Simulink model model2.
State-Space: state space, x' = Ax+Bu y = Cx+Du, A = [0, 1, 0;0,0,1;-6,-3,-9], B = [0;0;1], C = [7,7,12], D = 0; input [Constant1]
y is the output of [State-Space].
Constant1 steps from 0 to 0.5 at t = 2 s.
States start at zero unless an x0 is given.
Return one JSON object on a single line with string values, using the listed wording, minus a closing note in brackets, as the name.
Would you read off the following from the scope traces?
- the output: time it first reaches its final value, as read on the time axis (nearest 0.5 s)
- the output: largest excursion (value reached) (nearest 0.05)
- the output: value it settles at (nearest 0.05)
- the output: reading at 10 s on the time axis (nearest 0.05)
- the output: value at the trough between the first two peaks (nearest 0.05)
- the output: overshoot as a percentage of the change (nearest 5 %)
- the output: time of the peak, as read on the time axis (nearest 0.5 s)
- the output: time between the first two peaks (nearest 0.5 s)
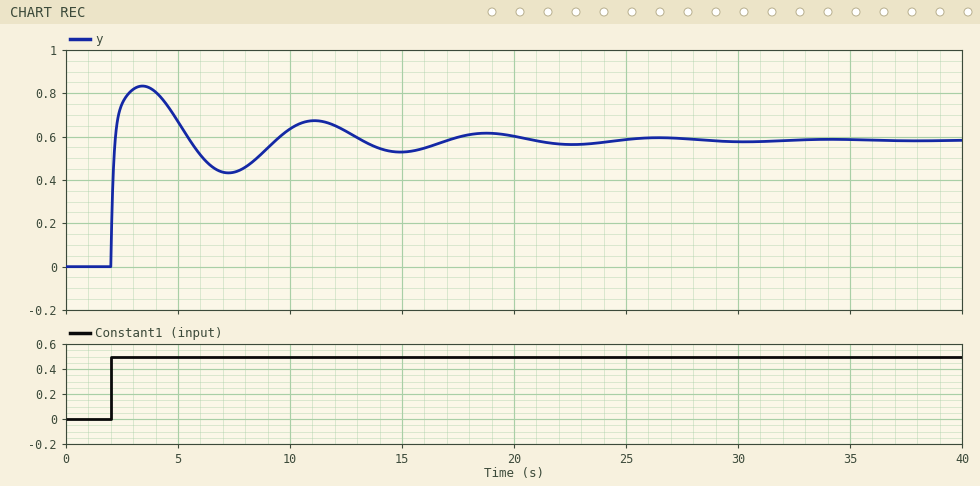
{"the output: time it first reaches its final value, as read on the time axis": "2.0 s", "the output: largest excursion (value reached)": "0.85", "the output: value it settles at": "0.60", "the output: reading at 10 s on the time axis": "0.65", "the output: value at the trough between the first two peaks": "0.45", "the output: overshoot as a percentage of the change": "45 %", "the output: time of the peak, as read on the time axis": "3.5 s", "the output: time between the first two peaks": "7.5 s"}
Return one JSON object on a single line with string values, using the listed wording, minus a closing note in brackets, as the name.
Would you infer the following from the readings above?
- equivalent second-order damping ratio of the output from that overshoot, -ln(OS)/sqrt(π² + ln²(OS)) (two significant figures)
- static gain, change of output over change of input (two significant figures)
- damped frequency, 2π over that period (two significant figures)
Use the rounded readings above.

{"equivalent second-order damping ratio of the output from that overshoot, -ln(OS)/sqrt(π² + ln²(OS))": "0.25", "static gain, change of output over change of input": "1.2", "damped frequency, 2π over that period": "0.84 rad/s"}
